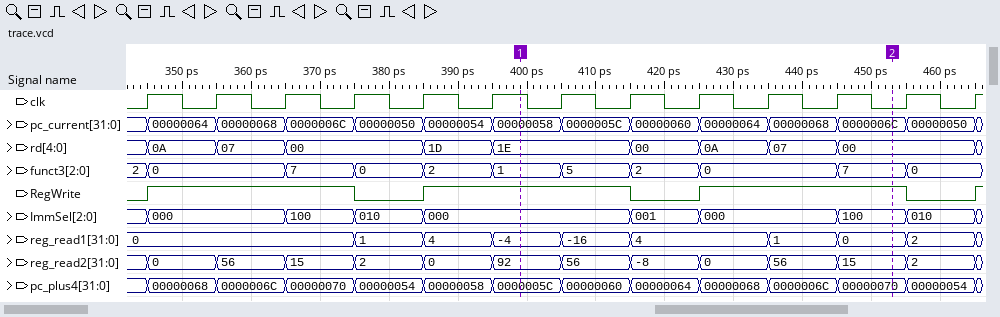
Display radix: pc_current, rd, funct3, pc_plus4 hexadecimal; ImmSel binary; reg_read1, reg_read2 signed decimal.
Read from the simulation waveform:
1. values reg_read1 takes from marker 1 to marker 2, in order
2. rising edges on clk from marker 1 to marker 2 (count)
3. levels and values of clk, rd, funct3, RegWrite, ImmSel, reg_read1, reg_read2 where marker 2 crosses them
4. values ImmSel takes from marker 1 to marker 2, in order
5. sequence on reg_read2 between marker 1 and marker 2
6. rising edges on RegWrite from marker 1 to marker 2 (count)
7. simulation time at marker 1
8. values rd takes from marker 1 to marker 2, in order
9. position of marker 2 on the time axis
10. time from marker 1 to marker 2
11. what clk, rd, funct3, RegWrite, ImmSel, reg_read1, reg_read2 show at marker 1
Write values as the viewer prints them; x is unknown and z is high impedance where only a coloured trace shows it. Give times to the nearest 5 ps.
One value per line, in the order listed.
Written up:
-4, -16, 4, 1, 0
5
clk=0, rd=00, funct3=7, RegWrite=1, ImmSel=100, reg_read1=0, reg_read2=15
000, 001, 000, 100
92, 56, -8, 0, 56, 15
1
400 ps
1E, 00, 0A, 07, 00
455 ps
55 ps
clk=1, rd=1E, funct3=1, RegWrite=1, ImmSel=000, reg_read1=-4, reg_read2=92
